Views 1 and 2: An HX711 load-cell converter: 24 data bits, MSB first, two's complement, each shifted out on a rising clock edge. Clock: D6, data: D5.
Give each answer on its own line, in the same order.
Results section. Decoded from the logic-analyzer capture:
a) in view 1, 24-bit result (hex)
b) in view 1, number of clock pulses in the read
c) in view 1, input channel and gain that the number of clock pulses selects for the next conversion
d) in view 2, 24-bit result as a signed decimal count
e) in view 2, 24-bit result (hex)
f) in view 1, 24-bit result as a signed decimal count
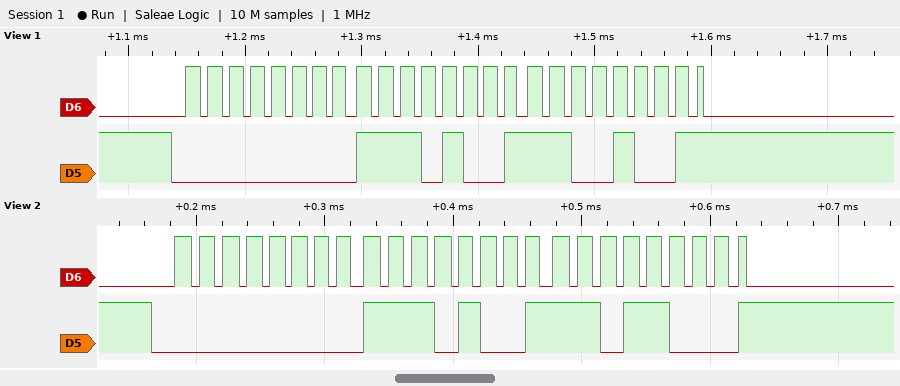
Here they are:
0x00E9C9
25
channel A, gain 128
59864
0x00E9D8
59849
